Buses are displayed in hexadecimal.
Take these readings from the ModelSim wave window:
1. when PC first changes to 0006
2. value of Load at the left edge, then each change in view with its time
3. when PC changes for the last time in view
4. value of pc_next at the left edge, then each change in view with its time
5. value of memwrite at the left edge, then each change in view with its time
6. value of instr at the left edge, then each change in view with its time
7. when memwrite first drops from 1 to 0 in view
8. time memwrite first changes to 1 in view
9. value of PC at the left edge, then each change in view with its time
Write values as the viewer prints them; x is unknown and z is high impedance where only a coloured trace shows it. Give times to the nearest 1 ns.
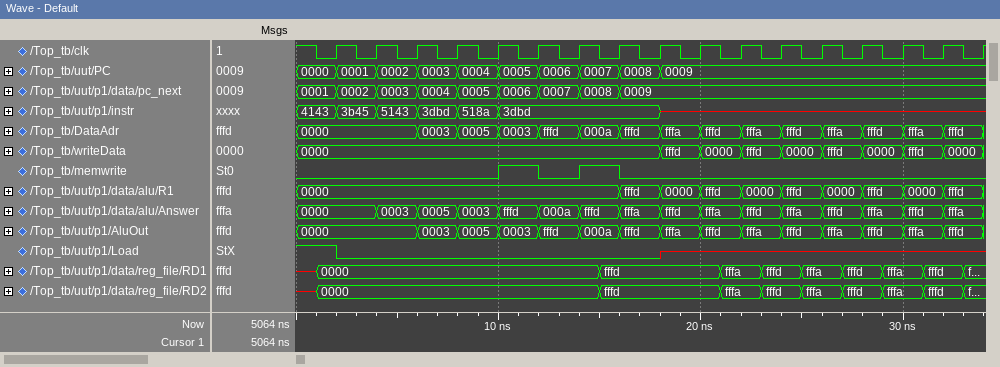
12 ns
1, 0 at 2 ns, x at 18 ns
18 ns
0001, 0002 at 2 ns, 0003 at 4 ns, 0004 at 6 ns, 0005 at 8 ns, 0006 at 10 ns, 0007 at 12 ns, 0008 at 14 ns, 0009 at 16 ns
0, 1 at 10 ns, 0 at 12 ns, 1 at 14 ns, 0 at 16 ns
4143, 3b45 at 2 ns, 5143 at 4 ns, 3dbd at 6 ns, 518a at 8 ns, 3dbd at 10 ns, x at 18 ns
12 ns
10 ns
0000, 0001 at 2 ns, 0002 at 4 ns, 0003 at 6 ns, 0004 at 8 ns, 0005 at 10 ns, 0006 at 12 ns, 0007 at 14 ns, 0008 at 16 ns, 0009 at 18 ns
